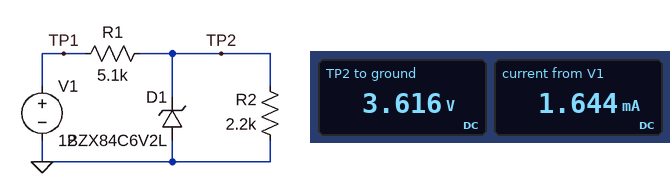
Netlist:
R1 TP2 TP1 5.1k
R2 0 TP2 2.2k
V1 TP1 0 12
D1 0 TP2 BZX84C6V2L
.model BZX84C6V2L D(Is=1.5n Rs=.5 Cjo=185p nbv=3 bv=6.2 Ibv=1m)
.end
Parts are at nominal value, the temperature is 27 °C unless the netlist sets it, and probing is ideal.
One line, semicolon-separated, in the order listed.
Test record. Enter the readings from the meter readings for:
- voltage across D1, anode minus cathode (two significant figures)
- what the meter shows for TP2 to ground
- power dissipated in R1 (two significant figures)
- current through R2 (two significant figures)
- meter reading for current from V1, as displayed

-3.6 V; 3.616 V; 14 mW; 1.6 mA; 1.644 mA
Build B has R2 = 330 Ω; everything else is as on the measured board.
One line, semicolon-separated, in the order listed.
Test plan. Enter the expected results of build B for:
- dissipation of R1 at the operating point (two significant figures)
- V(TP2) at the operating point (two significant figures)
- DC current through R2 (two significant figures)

25 mW; 730 mV; 2.2 mA
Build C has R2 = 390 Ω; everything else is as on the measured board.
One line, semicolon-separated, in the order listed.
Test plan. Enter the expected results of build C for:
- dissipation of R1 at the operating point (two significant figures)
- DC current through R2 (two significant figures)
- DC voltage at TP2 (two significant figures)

24 mW; 2.2 mA; 850 mV
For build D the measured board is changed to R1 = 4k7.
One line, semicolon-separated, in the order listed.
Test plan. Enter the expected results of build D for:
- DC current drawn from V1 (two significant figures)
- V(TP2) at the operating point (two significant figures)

1.7 mA; 3.8 V
